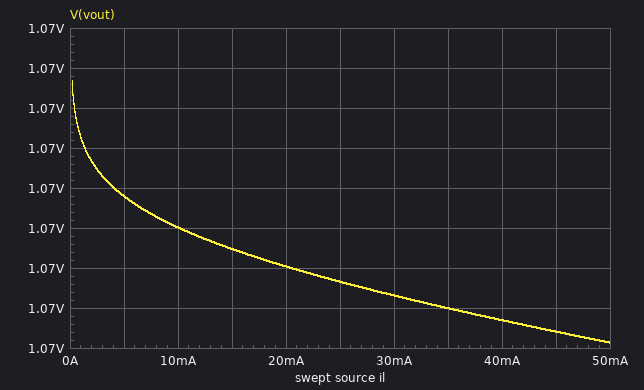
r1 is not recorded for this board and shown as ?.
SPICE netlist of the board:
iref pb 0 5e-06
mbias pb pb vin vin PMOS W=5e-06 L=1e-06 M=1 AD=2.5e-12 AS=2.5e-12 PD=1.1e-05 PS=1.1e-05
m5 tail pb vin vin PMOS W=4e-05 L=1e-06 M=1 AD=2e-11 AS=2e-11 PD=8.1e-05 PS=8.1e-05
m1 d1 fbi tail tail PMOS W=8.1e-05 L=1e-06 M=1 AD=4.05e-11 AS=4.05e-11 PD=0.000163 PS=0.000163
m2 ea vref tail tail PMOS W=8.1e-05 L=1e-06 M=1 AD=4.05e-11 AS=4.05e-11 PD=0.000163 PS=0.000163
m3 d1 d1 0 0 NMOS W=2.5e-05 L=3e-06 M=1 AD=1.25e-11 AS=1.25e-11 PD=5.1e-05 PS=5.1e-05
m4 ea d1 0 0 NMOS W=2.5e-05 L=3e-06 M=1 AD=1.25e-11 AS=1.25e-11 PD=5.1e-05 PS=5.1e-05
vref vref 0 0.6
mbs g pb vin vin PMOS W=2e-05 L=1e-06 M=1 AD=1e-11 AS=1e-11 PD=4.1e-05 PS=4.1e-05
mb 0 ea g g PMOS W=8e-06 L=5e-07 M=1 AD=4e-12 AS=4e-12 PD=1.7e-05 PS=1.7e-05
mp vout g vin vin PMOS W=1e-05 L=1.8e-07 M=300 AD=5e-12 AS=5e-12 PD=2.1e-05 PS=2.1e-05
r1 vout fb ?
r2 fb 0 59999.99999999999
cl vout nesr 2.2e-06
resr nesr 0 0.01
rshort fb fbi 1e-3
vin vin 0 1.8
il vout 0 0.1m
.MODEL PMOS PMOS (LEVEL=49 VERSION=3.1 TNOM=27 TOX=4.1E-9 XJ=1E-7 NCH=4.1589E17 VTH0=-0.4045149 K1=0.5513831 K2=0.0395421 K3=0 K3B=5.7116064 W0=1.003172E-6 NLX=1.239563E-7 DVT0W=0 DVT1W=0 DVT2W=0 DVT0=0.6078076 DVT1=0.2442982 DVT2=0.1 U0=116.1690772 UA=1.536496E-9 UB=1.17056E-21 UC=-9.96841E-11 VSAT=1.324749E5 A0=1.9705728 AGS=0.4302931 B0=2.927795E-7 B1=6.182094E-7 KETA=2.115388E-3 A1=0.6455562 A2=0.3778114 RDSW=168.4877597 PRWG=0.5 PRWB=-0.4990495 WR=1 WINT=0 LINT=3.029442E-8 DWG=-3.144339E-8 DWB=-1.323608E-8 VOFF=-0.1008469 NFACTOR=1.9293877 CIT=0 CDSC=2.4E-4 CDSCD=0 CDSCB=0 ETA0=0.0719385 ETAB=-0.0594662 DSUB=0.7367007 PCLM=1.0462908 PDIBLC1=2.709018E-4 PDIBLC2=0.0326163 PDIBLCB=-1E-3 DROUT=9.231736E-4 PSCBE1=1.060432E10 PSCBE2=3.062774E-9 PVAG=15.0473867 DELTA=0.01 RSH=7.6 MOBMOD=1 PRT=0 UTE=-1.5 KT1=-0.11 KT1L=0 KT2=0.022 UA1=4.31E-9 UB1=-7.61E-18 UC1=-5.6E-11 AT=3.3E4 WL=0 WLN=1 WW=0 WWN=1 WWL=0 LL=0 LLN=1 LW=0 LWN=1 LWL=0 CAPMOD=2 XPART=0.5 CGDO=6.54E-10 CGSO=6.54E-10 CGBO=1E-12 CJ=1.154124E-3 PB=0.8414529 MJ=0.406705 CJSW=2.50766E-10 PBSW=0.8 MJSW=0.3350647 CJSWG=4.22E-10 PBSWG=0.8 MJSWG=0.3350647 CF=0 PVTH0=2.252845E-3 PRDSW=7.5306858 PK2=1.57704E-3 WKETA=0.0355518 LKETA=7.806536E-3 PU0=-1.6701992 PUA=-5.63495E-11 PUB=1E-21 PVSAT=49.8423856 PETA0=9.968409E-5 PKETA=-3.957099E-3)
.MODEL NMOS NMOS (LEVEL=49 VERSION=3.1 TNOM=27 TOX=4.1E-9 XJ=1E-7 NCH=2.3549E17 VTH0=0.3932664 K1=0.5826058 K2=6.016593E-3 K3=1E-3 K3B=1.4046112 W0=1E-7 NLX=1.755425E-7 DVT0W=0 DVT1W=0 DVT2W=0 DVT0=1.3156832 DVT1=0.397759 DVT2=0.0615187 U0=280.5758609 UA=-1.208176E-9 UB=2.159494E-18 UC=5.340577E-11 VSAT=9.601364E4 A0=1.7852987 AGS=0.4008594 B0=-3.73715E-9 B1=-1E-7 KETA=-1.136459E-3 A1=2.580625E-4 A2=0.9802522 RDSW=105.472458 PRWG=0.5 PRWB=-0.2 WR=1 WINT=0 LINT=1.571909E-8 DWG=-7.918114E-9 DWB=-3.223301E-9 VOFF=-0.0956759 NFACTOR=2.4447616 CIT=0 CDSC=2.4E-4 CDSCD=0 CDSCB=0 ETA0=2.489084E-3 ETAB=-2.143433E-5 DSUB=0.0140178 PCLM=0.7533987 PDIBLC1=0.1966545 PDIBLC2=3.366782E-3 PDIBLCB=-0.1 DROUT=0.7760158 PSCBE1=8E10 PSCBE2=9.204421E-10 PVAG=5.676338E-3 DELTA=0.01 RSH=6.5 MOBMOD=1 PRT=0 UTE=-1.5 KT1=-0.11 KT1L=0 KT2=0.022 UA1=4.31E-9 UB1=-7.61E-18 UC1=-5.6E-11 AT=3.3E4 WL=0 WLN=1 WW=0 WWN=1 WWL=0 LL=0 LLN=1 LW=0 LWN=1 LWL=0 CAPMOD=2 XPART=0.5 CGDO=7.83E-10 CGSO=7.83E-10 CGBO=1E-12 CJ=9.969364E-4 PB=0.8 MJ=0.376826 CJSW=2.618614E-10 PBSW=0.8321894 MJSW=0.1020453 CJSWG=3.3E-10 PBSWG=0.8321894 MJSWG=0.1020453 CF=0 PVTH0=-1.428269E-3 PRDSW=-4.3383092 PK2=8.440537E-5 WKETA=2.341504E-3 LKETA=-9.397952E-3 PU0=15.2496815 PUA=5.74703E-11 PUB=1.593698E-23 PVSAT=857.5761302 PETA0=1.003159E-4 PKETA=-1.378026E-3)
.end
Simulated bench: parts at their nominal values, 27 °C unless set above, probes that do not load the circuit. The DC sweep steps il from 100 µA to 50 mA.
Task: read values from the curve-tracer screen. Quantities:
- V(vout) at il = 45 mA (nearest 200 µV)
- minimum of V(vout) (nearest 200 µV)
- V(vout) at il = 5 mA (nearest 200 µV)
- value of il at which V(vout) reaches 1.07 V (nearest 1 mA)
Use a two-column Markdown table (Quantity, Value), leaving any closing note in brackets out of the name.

| Quantity | Value |
|---|---|
| V(vout) at il = 45 mA | 1.0674 V |
| minimum of V(vout) | 1.0672 V |
| V(vout) at il = 5 mA | 1.0708 V |
| value of il at which V(vout) reaches 1.07 V | 10 mA |
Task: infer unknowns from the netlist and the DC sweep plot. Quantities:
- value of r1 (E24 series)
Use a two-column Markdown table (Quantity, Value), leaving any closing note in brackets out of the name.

| Quantity | Value |
|---|---|
| value of r1 | 47 kΩ |
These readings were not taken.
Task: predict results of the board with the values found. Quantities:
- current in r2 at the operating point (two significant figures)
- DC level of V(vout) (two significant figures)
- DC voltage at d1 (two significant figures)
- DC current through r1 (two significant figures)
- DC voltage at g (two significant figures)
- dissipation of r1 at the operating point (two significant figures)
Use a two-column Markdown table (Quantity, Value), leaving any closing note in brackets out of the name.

| Quantity | Value |
|---|---|
| current in r2 at the operating point | 10 µA |
| DC level of V(vout) | 1.1 V |
| DC voltage at d1 | 560 mV |
| DC current through r1 | 10 µA |
| DC voltage at g | 1.4 V |
| dissipation of r1 at the operating point | 4.7 µW |
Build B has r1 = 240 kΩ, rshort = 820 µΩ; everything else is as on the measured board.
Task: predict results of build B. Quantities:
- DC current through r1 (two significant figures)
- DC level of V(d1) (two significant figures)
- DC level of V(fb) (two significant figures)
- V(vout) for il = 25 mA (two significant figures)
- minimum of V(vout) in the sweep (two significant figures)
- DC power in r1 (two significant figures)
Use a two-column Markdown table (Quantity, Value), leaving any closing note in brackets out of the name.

| Quantity | Value |
|---|---|
| DC current through r1 | 6.0 µA |
| DC level of V(d1) | 620 mV |
| DC level of V(fb) | 360 mV |
| V(vout) for il = 25 mA | 1.8 V |
| minimum of V(vout) in the sweep | 1.7 V |
| DC power in r1 | 8.6 µW |
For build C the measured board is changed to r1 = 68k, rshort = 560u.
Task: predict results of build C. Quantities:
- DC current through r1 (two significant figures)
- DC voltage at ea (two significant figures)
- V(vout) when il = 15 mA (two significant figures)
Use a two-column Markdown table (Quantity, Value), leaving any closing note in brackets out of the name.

| Quantity | Value |
|---|---|
| DC current through r1 | 10 µA |
| DC voltage at ea | 780 mV |
| V(vout) when il = 15 mA | 1.3 V |
